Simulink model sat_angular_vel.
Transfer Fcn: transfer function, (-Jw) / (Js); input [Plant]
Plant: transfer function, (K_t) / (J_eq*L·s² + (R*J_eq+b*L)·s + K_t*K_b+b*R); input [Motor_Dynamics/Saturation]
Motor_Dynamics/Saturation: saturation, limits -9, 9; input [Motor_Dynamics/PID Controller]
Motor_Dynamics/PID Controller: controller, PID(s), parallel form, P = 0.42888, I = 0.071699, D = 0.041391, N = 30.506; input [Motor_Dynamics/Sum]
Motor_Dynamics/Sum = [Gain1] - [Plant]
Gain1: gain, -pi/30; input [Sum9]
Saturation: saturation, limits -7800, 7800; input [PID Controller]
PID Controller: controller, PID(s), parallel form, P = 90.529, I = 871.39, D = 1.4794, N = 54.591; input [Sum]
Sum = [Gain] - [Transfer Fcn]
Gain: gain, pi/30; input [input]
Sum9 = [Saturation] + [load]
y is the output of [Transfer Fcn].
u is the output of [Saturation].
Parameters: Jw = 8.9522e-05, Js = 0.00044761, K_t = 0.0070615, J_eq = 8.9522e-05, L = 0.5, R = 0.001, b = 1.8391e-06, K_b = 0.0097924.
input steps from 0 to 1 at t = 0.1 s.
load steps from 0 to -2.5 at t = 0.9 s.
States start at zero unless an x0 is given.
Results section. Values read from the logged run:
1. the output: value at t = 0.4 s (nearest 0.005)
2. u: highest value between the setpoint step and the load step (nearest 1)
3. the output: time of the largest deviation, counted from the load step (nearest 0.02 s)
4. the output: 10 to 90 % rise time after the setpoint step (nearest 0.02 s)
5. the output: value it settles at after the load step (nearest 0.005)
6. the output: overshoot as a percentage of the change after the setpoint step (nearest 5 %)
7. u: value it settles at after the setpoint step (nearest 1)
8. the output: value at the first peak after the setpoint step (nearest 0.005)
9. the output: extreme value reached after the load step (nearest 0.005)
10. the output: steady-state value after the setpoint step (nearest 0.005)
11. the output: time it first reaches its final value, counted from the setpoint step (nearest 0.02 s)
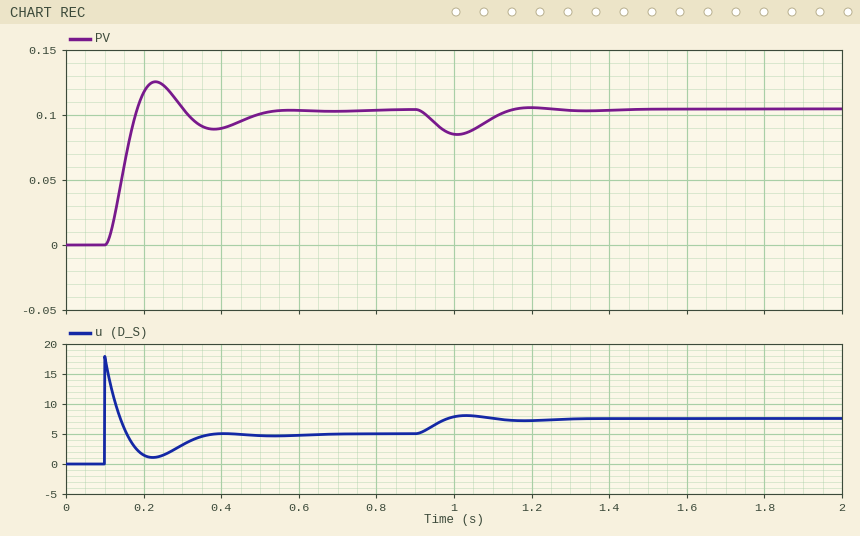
0.090
18
0.10 s
0.06 s
0.105
20 %
5
0.125
0.085
0.105
0.08 s
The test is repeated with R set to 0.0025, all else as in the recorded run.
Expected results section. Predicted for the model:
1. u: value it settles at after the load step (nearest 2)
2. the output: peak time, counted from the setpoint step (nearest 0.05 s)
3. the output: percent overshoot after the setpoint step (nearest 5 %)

8
0.15 s
20 %
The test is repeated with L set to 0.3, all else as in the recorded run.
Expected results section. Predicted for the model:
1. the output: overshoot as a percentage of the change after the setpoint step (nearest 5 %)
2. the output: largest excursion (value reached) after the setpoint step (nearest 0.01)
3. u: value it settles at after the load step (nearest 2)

15 %
0.12
8
